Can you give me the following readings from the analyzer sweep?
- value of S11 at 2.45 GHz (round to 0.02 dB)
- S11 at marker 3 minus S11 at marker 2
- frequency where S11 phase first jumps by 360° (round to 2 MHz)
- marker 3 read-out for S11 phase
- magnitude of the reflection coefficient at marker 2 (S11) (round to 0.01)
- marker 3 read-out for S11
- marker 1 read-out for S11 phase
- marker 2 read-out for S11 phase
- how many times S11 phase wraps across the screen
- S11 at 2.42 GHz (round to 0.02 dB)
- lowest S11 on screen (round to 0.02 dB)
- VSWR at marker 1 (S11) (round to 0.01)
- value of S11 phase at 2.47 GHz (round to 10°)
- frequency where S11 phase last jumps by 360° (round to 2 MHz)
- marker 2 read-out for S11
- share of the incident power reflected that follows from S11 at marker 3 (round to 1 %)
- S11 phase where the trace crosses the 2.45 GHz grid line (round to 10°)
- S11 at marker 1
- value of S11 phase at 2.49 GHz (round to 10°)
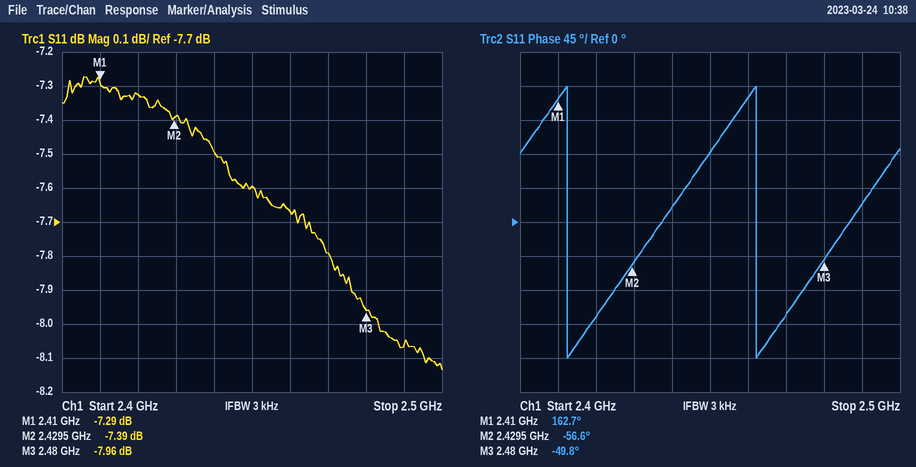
-7.60 dB
-0.57 dB
2.412 GHz
-49.8°
0.43
-7.96 dB
162.7°
-56.6°
2
-7.32 dB
-8.14 dB
2.52
-120°
2.462 GHz
-7.39 dB
16 %
90°
-7.29 dB
20°
